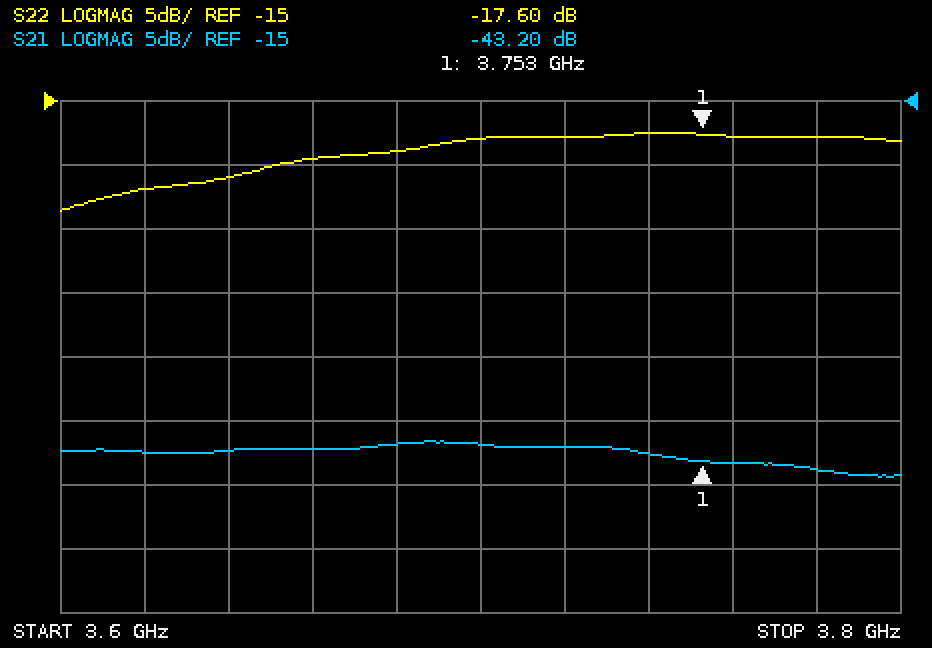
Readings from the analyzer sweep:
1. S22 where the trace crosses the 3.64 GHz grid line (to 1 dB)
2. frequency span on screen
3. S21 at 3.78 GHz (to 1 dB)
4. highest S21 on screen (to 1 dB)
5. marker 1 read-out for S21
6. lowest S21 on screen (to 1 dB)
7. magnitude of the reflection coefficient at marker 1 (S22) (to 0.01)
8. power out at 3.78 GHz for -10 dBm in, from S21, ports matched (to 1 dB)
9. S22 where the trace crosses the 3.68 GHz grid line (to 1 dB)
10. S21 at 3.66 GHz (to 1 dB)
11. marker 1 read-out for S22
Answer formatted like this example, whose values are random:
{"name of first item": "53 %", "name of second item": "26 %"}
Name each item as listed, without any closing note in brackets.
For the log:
{"S22 where the trace crosses the 3.64 GHz grid line": "-21 dB", "frequency span on screen": "200 MHz", "S21 at 3.78 GHz": "-44 dB", "highest S21 on screen": "-42 dB", "marker 1 read-out for S21": "-43.20 dB", "lowest S21 on screen": "-44 dB", "magnitude of the reflection coefficient at marker 1 (S22)": "0.13", "power out at 3.78 GHz for -10 dBm in, from S21, ports matched": "-54 dBm", "S22 where the trace crosses the 3.68 GHz grid line": "-19 dB", "S21 at 3.66 GHz": "-42 dB", "marker 1 read-out for S22": "-17.60 dB"}
